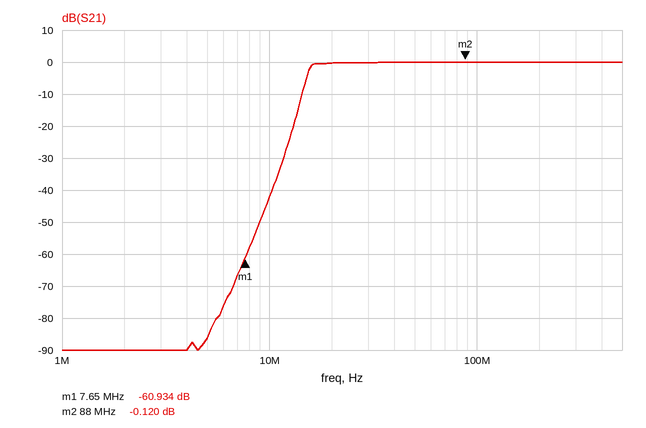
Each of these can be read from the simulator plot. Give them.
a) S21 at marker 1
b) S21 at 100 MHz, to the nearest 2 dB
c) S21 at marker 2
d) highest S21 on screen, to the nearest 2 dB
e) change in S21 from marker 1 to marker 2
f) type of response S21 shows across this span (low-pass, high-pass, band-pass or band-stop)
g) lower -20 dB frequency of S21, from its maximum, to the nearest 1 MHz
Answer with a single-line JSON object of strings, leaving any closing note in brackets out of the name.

{"S21 at marker 1": "-60.934 dB", "S21 at 100 MHz, to the nearest 2 dB": "0 dB", "S21 at marker 2": "-0.120 dB", "highest S21 on screen, to the nearest 2 dB": "0 dB", "change in S21 from marker 1 to marker 2": "60.814 dB", "type of response S21 shows across this span": "high-pass", "lower -20 dB frequency of S21, from its maximum, to the nearest 1 MHz": "13 MHz"}
